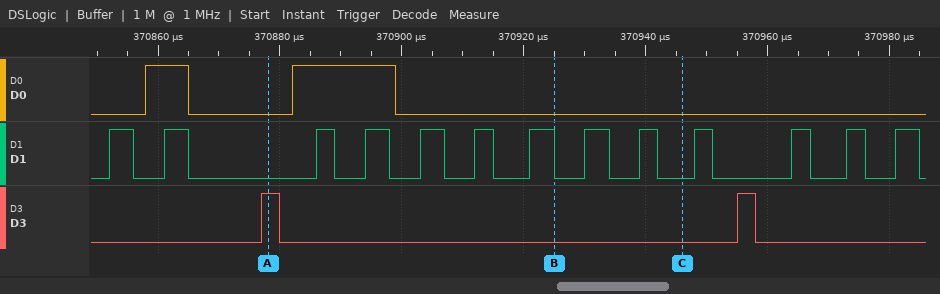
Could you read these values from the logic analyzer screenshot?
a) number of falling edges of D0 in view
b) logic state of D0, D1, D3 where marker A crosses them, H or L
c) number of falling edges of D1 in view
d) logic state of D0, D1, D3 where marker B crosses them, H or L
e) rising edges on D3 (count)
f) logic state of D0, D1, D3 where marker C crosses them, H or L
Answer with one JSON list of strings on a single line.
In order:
["2", "D0=L, D1=L, D3=H", "13", "D0=L, D1=L, D3=L", "2", "D0=L, D1=L, D3=L"]
